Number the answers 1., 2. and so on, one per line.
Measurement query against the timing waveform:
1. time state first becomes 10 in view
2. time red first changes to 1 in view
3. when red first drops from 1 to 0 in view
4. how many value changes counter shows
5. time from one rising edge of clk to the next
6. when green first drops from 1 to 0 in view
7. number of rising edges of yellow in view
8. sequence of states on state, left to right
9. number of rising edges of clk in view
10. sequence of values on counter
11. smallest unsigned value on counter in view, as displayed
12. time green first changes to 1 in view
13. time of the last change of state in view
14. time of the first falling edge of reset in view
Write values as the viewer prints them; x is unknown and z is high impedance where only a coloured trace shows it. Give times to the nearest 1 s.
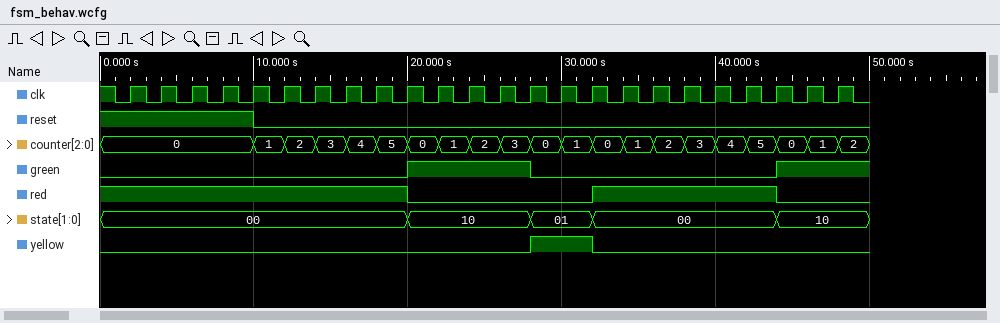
1. 20 s
2. 32 s
3. 20 s
4. 20
5. 2 s
6. 28 s
7. 1
8. 00, 10, 01, 00, 10
9. 24
10. 0, 1, 2, 3, 4, 5, 0, 1, 2, 3, 0, 1, 0, 1, 2, 3, 4, 5, 0, 1, 2
11. 0
12. 20 s
13. 44 s
14. 10 s
